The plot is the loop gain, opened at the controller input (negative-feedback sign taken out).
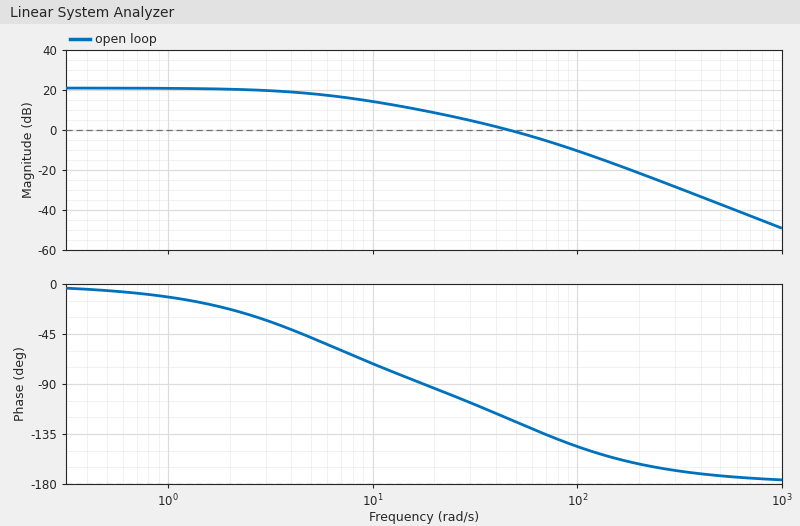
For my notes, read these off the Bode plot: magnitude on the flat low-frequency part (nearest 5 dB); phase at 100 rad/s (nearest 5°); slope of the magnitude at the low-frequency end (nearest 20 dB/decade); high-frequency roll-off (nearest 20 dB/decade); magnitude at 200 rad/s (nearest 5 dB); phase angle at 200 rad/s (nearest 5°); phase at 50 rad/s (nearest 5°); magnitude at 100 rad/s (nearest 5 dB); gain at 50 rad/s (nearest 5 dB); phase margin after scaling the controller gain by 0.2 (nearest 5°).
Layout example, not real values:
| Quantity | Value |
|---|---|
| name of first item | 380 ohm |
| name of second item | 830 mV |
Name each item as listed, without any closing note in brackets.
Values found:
| Quantity | Value |
|---|---|
| magnitude on the flat low-frequency part | 20 dB |
| phase at 100 rad/s | -145° |
| slope of the magnitude at the low-frequency end | 0 dB/decade |
| high-frequency roll-off | -40 dB/decade |
| magnitude at 200 rad/s | -20 dB |
| phase angle at 200 rad/s | -160° |
| phase at 50 rad/s | -125° |
| magnitude at 100 rad/s | -10 dB |
| gain at 50 rad/s | 0 dB |
| phase margin after scaling the controller gain by 0.2 | 105° |
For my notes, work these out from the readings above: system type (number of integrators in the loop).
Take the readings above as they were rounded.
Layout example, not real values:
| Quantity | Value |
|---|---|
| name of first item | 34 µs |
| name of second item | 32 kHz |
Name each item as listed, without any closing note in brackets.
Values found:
| Quantity | Value |
|---|---|
| system type | 0 |
